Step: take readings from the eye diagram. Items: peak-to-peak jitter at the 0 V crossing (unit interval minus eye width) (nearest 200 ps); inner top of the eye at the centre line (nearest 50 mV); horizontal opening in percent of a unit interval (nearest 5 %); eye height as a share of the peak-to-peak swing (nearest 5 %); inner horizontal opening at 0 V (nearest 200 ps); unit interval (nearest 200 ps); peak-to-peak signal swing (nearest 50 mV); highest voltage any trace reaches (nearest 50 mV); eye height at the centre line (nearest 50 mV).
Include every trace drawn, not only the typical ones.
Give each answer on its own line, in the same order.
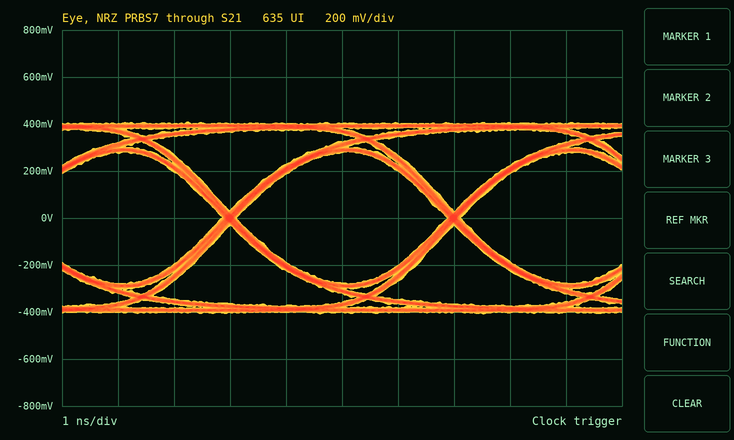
200 ps
300 mV
95 %
70 %
3.8 ns
4.0 ns
800 mV
400 mV
550 mV
